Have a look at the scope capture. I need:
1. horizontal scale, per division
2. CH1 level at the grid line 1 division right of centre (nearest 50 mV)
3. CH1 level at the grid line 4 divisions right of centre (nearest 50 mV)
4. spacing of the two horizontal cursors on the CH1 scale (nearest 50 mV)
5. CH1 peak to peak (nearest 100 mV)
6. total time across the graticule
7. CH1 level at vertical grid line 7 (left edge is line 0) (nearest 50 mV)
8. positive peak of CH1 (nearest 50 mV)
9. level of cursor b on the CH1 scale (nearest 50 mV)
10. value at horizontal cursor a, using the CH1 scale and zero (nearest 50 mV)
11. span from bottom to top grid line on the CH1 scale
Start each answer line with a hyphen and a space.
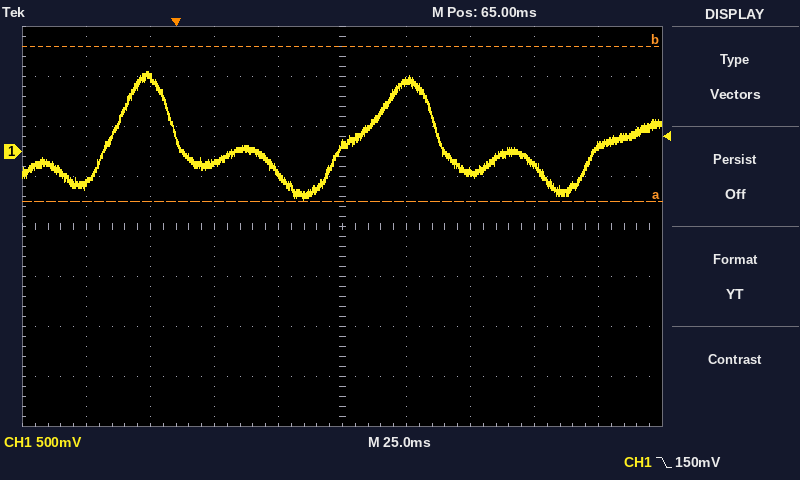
- 25 ms
- 700 mV
- 50 mV
- 1.55 V
- 1.30 V
- 250 ms
- -200 mV
- 800 mV
- 1.05 V
- -500 mV
- 4 V
